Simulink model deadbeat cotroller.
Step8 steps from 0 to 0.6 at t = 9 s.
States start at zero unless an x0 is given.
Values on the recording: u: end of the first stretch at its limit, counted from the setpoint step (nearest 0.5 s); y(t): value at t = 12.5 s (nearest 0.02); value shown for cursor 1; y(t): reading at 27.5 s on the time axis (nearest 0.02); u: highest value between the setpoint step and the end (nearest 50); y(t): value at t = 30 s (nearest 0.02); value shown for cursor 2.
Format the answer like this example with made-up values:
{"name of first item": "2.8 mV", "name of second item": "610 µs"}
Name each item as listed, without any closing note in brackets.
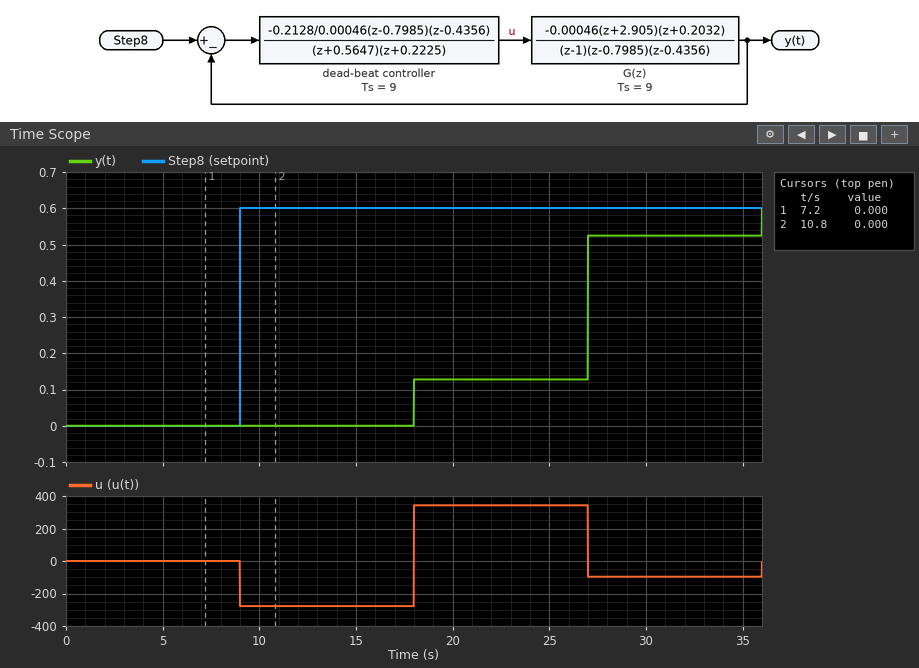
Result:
{"u: end of the first stretch at its limit, counted from the setpoint step": "9.0 s", "y(t): value at t = 12.5 s": "0.00", "value shown for cursor 1": "0.000", "y(t): reading at 27.5 s on the time axis": "0.52", "u: highest value between the setpoint step and the end": "350", "y(t): value at t = 30 s": "0.52", "value shown for cursor 2": "0.000"}
